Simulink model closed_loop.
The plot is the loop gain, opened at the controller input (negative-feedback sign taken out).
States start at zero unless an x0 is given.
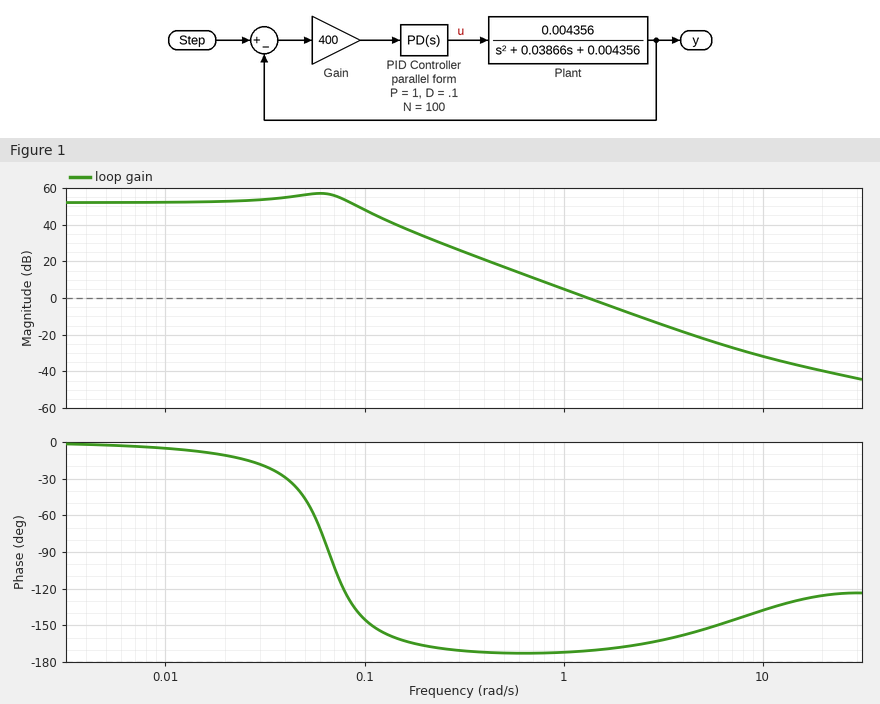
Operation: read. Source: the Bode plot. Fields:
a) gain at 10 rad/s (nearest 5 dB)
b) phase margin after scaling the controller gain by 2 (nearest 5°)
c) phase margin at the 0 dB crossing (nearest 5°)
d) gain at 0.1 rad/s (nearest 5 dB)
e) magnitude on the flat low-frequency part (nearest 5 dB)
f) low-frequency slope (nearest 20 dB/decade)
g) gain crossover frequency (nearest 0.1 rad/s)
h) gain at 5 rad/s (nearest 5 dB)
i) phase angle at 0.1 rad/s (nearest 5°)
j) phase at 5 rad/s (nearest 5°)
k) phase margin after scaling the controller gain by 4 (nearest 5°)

-30 dB
10°
10°
50 dB
50 dB
0 dB/decade
1.3 rad/s
-20 dB
-145°
-155°
15°
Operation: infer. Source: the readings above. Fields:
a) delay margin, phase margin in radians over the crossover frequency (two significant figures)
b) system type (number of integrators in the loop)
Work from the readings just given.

0.13 s
0
